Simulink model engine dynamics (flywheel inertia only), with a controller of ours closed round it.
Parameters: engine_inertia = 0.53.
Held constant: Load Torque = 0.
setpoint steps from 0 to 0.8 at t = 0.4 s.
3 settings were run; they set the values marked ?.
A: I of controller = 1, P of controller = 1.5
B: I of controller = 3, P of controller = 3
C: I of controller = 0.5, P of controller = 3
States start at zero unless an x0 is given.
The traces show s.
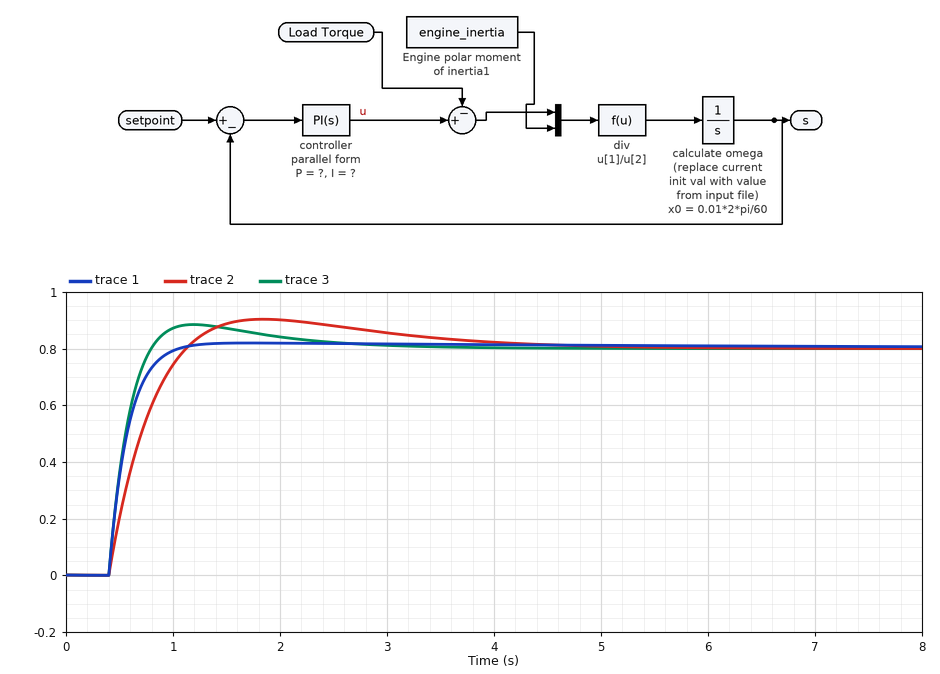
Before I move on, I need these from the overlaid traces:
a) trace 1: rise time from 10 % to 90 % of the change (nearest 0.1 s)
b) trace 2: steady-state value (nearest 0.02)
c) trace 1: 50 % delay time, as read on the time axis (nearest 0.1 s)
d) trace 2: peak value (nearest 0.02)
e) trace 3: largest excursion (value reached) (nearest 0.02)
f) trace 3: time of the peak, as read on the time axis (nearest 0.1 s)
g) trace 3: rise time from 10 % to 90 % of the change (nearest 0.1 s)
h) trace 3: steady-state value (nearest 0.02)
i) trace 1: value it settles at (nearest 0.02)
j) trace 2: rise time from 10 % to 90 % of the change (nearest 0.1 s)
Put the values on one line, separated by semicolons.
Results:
0.4 s; 0.80; 0.5 s; 0.90; 0.88; 1.2 s; 0.3 s; 0.80; 0.80; 0.5 s
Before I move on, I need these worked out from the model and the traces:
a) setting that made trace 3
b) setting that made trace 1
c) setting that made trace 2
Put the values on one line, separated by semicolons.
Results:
B; C; A
